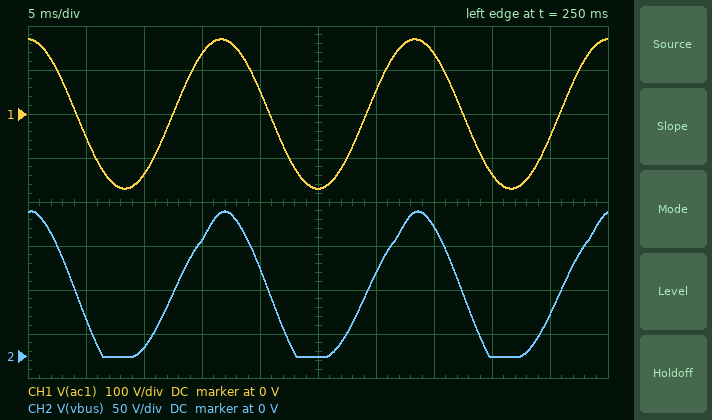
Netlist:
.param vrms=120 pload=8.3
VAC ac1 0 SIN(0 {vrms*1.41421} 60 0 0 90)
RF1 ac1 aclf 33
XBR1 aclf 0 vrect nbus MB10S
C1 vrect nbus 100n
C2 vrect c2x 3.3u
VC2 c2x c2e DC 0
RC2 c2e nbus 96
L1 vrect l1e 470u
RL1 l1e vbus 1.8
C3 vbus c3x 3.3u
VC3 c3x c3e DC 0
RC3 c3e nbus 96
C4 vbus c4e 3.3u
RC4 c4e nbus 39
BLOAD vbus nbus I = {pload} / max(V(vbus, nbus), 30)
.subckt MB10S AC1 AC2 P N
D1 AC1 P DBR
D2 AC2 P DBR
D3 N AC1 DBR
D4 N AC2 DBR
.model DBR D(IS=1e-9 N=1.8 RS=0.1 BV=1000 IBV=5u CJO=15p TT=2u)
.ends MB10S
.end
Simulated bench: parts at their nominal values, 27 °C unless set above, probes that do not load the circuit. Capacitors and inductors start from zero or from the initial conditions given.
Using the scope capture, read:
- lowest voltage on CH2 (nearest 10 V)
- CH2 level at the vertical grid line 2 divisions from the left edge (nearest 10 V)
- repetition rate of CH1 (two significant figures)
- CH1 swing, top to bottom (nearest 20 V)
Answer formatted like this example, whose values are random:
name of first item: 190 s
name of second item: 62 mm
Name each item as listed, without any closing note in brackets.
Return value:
lowest voltage on CH2: 0 V
CH2 level at the vertical grid line 2 divisions from the left edge: 10 V
repetition rate of CH1: 60 Hz
CH1 swing, top to bottom: 340 V
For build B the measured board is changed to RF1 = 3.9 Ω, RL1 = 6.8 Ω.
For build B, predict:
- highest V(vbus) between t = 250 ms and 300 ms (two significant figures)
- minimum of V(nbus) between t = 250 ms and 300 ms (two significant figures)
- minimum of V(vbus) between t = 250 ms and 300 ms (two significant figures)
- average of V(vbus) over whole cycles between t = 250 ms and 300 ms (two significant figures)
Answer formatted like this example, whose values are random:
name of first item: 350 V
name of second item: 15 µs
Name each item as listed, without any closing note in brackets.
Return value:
highest V(vbus) between t = 250 ms and 300 ms: 170 V
minimum of V(nbus) between t = 250 ms and 300 ms: -170 V
minimum of V(vbus) between t = 250 ms and 300 ms: -2.5 V
average of V(vbus) over whole cycles between t = 250 ms and 300 ms: 75 V
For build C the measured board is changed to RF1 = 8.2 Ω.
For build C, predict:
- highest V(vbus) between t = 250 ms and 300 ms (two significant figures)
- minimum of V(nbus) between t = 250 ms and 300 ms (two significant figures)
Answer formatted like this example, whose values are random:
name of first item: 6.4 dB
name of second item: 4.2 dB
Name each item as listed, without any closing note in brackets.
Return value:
highest V(vbus) between t = 250 ms and 300 ms: 170 V
minimum of V(nbus) between t = 250 ms and 300 ms: -170 V
